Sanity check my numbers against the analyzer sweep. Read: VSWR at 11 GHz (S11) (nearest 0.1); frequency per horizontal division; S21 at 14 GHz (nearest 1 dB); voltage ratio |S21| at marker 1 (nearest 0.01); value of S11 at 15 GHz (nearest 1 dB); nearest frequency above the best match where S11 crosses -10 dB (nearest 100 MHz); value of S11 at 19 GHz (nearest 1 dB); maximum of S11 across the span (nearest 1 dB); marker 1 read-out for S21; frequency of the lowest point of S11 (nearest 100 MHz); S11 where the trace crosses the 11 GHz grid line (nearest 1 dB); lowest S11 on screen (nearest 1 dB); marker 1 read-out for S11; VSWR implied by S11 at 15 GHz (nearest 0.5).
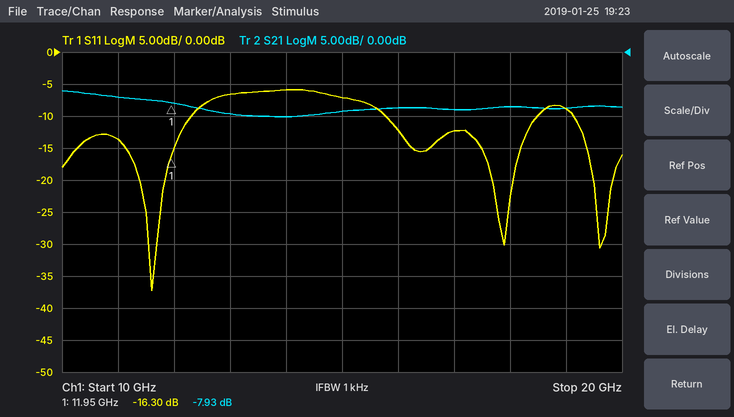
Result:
1.5
1 GHz
-10 dB
0.40
-7 dB
12.3 GHz
-9 dB
-6 dB
-7.93 dB
11.6 GHz
-14 dB
-37 dB
-16.30 dB
2.5
